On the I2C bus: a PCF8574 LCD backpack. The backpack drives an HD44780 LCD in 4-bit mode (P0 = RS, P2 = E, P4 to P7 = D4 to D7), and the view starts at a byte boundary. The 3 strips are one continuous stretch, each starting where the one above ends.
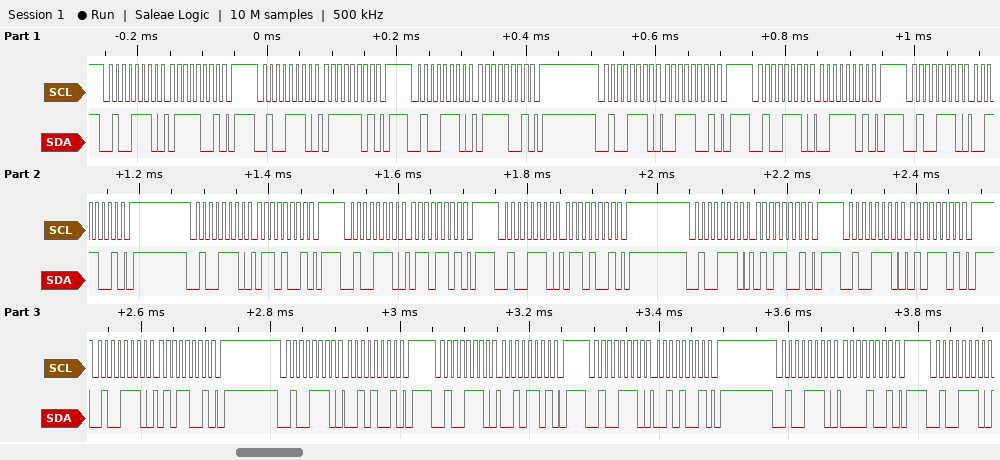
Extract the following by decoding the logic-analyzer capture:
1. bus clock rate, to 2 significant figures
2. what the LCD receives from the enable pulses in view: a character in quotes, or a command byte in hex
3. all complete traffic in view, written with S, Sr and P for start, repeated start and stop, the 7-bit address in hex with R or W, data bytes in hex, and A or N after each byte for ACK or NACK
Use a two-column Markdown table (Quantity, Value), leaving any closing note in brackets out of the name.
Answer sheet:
| Quantity | Value |
|---|---|
| bus clock rate, to 2 significant figures | 100 kHz |
| what the LCD receives from the enable pulses in view: a character in quotes, or a command byte in hex | 's' 'e' |
| all complete traffic in view, written with S, Sr and P for start, repeated start and stop, the 7-bit address in hex with R or W, data bytes in hex, and A or N after each byte for ACK or NACK | S 27W A 79 A P S 27W A 7D A P S 27W A 79 A P S 27W A 39 A P S 27W A 3D A P S 27W A 39 A P S 27W A 69 A P S 27W A 6D A P S 27W A 69 A P S 27W A 59 A P S 27W A 5D A P S 27W A 59 A P S 27W A 29 A P S 27W A 2D A P S 27W A 29 A P S 27W A 09 A P S 27W A |
